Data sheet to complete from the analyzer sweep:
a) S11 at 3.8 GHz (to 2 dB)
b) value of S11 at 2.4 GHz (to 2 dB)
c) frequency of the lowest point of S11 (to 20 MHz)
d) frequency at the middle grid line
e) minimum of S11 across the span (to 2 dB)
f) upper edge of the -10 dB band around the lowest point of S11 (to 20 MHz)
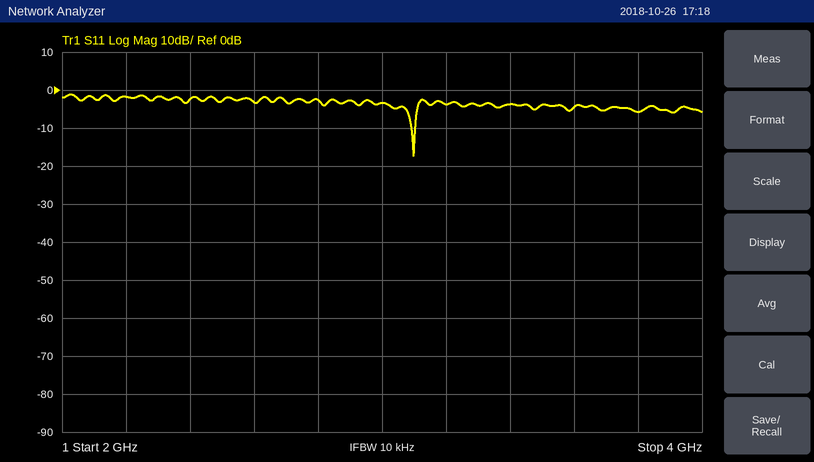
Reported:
-6 dB
-2 dB
3.10 GHz
3 GHz
-18 dB
3.10 GHz
